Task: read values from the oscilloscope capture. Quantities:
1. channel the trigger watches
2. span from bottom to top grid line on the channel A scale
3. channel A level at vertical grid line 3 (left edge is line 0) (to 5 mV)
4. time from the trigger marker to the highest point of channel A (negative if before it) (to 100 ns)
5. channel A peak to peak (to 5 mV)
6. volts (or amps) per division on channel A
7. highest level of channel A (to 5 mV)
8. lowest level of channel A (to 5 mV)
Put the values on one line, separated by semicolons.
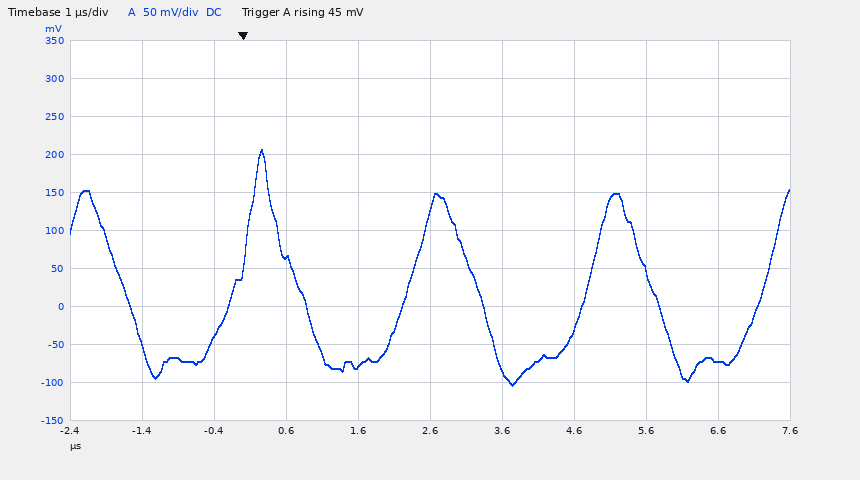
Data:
channel A; 500 mV; 65 mV; +300 ns; 310 mV; 50 mV; 205 mV; -105 mV
